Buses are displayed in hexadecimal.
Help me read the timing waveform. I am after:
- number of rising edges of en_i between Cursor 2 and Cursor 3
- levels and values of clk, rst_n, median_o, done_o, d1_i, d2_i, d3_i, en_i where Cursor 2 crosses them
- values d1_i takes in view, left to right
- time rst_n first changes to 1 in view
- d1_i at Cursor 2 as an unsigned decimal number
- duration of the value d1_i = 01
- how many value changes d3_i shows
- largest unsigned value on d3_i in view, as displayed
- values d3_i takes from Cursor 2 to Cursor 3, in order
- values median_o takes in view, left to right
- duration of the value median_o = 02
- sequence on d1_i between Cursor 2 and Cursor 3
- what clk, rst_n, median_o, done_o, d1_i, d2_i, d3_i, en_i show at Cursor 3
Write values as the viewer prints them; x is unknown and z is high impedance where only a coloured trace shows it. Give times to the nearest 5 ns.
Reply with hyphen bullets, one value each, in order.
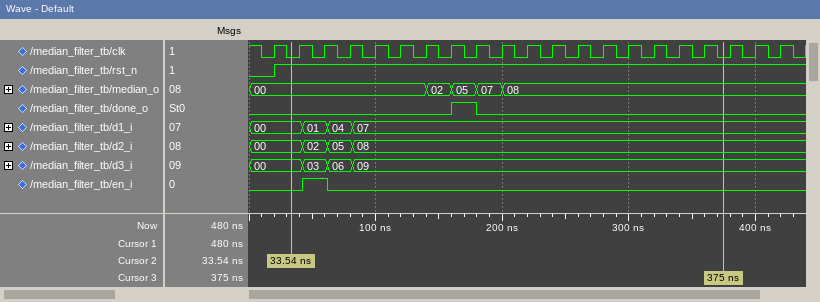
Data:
- 1
- clk=0, rst_n=1, median_o=00, done_o=0, d1_i=00, d2_i=00, d3_i=00, en_i=0
- 00, 01, 04, 07
- 20 ns
- 0
- 20 ns
- 3
- 09
- 00, 03, 06, 09
- 00, 02, 05, 07, 08
- 20 ns
- 00, 01, 04, 07
- clk=0, rst_n=1, median_o=08, done_o=0, d1_i=07, d2_i=08, d3_i=09, en_i=0
